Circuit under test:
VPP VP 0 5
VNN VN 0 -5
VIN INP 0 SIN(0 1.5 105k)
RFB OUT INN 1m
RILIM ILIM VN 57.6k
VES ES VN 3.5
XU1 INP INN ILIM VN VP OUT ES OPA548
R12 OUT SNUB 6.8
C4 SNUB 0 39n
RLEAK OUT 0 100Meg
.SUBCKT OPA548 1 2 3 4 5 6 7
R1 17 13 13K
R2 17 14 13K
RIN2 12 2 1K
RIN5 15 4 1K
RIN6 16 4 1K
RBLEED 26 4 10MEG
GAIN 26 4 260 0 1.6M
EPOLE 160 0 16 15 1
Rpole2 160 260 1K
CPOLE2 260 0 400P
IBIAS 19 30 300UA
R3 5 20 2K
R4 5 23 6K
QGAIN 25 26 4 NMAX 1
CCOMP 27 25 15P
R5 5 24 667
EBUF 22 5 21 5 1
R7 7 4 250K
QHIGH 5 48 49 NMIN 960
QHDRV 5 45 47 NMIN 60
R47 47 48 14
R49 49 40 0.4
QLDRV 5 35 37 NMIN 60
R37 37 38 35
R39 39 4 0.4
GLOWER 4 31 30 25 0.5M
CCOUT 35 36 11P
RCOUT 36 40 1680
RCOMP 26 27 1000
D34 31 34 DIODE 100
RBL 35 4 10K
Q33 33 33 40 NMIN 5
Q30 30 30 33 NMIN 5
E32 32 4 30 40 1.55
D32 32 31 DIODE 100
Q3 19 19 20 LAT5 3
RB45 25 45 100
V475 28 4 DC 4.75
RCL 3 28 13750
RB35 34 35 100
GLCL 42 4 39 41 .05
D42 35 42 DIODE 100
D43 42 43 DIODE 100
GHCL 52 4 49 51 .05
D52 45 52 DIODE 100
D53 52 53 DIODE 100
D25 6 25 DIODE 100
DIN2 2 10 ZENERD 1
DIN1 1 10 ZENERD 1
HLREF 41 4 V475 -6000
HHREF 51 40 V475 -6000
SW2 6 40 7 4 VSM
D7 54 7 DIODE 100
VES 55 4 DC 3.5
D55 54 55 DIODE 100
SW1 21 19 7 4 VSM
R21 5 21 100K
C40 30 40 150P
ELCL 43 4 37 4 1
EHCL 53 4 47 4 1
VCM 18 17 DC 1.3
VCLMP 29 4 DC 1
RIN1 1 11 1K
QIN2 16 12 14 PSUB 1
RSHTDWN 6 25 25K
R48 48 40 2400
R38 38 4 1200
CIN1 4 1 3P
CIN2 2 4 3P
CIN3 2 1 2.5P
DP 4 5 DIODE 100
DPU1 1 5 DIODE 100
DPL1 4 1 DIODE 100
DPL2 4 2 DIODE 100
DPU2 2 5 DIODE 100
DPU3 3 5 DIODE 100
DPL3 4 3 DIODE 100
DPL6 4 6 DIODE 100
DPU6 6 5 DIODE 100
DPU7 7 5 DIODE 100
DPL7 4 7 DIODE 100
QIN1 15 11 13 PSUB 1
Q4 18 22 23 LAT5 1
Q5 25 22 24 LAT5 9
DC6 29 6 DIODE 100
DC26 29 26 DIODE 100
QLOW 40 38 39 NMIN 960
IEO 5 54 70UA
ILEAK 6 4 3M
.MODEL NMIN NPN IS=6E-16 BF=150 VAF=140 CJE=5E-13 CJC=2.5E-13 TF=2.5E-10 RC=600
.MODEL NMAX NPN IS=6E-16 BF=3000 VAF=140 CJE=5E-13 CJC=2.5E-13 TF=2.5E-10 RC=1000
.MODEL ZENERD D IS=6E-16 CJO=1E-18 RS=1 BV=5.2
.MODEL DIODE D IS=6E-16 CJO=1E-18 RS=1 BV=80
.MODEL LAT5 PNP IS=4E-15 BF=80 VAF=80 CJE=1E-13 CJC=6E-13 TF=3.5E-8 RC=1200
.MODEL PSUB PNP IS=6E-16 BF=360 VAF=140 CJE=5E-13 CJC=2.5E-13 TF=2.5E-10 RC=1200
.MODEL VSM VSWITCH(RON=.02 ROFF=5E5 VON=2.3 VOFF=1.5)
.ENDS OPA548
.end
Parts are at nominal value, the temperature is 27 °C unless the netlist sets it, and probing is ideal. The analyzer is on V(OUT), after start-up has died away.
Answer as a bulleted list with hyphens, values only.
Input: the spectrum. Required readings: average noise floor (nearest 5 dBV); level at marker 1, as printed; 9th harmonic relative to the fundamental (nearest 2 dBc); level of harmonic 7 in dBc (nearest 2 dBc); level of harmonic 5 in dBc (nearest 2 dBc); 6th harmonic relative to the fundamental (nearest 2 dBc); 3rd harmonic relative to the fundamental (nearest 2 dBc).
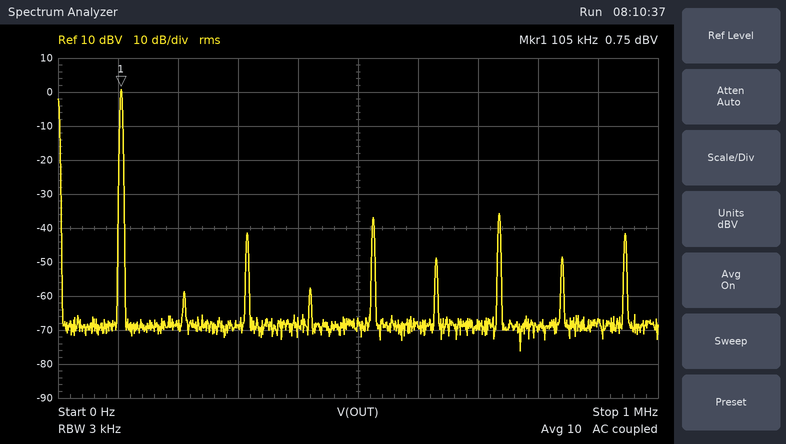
- -70 dBV
- 0.75 dBV
- -42 dBc
- -36 dBc
- -38 dBc
- -50 dBc
- -42 dBc
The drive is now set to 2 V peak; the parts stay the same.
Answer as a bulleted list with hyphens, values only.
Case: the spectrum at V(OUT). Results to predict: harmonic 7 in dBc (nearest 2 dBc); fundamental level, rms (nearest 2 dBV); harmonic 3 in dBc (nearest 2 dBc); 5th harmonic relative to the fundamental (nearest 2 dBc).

- -38 dBc
- 4 dBV
- -44 dBc
- -40 dBc
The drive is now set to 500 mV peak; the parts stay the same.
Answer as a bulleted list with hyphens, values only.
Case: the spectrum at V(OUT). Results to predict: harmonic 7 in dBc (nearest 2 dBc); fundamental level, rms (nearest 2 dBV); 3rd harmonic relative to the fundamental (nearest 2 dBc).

- -32 dBc
- -8 dBV
- -36 dBc
